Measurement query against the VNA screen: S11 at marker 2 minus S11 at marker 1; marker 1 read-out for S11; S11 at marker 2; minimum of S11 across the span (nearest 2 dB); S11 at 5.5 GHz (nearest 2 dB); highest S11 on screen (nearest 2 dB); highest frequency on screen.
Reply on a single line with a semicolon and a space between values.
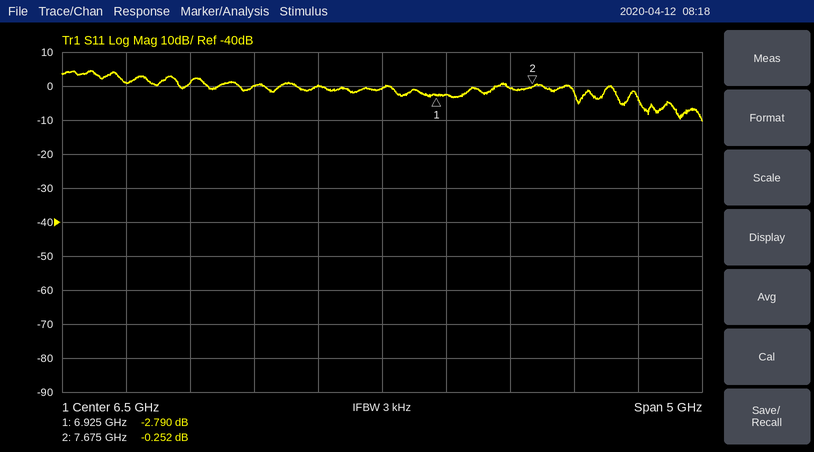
2.538 dB; -2.790 dB; -0.252 dB; -10 dB; 0 dB; 4 dB; 9 GHz
